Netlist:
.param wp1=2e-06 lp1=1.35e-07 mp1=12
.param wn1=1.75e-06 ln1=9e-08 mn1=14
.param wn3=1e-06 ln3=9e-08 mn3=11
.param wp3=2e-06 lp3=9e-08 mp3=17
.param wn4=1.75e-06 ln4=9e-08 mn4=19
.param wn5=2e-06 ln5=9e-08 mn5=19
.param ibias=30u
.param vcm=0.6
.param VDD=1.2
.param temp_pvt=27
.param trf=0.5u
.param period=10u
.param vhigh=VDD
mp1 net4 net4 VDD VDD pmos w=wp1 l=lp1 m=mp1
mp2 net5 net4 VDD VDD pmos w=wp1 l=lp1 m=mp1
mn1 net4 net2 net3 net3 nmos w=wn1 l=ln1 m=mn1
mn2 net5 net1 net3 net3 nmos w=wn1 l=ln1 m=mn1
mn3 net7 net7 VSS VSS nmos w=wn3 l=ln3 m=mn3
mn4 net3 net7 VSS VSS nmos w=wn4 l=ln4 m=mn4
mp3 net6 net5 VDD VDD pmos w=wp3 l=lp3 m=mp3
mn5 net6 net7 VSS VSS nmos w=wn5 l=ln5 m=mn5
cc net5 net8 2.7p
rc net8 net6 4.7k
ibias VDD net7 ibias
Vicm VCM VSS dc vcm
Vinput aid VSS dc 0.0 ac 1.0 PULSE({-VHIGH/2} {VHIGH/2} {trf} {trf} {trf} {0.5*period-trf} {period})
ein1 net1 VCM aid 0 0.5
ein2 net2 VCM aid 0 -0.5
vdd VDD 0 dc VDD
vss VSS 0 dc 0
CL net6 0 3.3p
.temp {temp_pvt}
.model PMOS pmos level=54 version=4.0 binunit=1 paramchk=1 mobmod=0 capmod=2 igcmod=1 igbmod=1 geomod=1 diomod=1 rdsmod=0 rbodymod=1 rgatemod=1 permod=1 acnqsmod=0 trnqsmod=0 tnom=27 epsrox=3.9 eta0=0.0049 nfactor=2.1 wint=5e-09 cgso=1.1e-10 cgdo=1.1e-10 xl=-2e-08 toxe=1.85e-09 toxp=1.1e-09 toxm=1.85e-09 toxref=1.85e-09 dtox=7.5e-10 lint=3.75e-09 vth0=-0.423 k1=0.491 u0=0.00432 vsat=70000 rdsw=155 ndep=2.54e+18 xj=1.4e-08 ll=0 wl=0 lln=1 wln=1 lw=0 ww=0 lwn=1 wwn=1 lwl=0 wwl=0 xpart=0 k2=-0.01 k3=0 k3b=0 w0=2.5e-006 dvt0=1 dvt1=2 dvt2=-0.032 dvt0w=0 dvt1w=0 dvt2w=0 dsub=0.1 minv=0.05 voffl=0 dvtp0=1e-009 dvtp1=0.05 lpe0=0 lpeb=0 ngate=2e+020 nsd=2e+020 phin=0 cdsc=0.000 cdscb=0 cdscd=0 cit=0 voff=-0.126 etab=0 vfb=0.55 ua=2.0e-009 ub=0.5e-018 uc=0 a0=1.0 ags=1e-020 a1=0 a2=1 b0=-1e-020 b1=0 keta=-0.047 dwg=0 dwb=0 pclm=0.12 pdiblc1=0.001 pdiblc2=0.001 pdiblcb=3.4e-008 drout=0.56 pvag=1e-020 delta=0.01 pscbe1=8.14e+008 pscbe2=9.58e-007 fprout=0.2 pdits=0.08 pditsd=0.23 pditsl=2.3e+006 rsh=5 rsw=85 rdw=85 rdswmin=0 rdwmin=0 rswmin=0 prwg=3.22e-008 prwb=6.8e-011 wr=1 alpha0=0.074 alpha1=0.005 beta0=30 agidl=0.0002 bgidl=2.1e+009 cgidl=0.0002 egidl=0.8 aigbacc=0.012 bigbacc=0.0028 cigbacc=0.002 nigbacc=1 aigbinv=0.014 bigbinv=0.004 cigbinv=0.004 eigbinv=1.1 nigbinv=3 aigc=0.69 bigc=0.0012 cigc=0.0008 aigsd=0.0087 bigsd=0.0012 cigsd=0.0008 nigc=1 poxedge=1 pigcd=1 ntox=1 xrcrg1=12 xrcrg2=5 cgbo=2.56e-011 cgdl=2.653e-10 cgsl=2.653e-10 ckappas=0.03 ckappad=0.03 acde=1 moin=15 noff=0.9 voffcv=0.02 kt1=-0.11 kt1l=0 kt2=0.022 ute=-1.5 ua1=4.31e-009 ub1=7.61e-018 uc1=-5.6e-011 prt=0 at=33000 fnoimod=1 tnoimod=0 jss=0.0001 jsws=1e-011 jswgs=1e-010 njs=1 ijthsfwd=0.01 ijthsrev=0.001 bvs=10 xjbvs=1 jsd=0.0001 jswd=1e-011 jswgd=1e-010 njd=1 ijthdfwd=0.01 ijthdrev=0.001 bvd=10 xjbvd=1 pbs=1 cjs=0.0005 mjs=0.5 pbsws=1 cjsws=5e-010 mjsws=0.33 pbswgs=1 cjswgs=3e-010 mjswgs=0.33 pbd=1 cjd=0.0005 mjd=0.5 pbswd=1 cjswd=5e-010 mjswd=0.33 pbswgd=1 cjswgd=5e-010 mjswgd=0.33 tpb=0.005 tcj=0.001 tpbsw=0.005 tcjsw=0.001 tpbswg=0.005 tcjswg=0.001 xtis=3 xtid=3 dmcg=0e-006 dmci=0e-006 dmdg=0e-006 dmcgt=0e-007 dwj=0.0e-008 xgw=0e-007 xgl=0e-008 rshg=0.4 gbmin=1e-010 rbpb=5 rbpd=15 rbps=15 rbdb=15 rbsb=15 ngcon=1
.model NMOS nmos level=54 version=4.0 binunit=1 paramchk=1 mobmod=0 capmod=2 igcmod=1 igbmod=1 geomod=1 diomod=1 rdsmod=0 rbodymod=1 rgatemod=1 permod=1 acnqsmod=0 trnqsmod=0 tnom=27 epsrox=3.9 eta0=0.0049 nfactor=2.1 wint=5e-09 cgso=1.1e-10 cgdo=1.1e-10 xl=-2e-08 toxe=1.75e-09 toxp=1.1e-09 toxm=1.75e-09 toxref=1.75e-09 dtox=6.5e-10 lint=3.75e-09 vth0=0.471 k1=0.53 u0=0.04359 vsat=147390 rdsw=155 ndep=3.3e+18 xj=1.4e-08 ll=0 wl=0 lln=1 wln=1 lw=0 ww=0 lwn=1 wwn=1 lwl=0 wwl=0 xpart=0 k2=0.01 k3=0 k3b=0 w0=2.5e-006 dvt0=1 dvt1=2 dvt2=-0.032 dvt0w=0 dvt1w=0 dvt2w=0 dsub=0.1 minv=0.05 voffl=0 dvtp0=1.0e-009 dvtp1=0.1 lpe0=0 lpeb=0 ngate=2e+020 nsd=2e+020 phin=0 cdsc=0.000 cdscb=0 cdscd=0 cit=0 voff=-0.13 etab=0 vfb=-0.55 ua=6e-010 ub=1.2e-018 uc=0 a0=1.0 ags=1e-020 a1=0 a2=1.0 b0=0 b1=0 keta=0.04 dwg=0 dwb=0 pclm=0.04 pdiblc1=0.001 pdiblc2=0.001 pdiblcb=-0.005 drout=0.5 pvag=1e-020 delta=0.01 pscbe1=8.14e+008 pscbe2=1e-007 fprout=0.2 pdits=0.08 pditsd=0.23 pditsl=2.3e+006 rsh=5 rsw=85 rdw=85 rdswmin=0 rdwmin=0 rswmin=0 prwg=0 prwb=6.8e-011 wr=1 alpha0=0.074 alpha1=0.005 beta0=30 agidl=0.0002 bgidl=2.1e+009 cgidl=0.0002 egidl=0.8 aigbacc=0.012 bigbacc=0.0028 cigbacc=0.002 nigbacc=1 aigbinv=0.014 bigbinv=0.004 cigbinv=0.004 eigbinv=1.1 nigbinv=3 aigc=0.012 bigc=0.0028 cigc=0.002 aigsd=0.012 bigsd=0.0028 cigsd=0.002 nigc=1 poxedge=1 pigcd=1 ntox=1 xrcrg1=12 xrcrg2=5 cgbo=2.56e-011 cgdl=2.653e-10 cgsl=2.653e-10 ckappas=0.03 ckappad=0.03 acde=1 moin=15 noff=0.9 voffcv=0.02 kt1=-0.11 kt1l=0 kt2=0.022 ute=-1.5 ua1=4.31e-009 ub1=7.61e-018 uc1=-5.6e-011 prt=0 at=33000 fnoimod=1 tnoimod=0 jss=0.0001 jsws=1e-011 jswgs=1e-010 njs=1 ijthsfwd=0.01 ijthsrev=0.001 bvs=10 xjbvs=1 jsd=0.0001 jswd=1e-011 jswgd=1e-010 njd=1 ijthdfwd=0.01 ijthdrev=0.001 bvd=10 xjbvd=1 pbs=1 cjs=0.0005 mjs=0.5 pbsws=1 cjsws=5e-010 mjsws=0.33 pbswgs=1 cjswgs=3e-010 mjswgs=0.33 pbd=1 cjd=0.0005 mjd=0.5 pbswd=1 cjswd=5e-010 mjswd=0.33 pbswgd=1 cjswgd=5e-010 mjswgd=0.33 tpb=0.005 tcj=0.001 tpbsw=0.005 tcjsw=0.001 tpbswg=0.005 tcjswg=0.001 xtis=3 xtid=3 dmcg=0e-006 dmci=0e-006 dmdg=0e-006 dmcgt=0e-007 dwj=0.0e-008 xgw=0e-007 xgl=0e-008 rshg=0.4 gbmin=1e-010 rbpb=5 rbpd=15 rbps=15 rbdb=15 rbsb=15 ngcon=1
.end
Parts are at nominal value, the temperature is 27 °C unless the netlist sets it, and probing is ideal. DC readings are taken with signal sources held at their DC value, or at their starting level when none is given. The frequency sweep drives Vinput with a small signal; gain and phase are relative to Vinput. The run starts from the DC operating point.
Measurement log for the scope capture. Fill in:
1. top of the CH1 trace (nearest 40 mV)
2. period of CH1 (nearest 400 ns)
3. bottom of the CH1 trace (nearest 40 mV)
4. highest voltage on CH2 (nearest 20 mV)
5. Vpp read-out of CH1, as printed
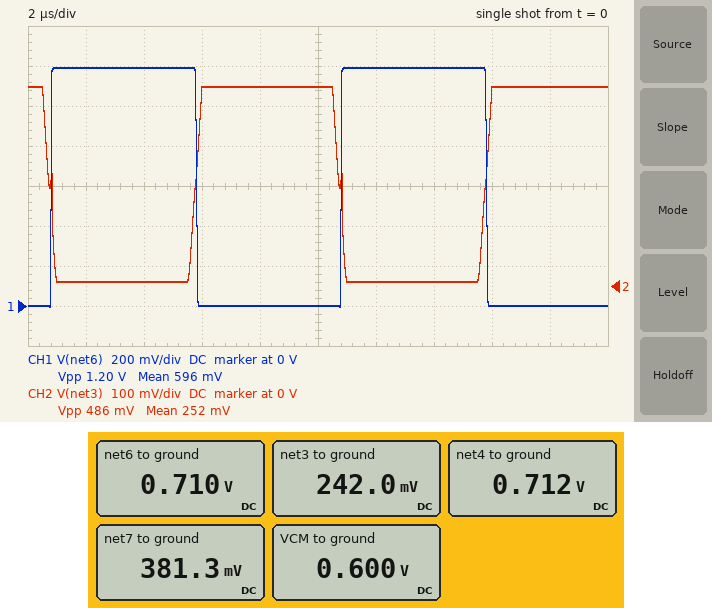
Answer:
1.20 V
10.0 µs
0 V
500 mV
1.20 V
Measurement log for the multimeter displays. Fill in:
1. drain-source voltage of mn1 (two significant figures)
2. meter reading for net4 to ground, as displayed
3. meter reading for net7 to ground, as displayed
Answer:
470 mV
0.712 V
381.3 mV
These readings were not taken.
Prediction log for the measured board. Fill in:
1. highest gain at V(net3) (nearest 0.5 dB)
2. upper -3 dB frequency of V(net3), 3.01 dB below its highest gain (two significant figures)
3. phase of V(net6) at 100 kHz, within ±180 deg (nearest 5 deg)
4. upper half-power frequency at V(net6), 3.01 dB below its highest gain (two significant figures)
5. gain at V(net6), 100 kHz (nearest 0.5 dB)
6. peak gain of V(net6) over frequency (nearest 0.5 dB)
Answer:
-9.0 dB
50 kHz
-65 deg
50 kHz
52.5 dB
59.5 dB
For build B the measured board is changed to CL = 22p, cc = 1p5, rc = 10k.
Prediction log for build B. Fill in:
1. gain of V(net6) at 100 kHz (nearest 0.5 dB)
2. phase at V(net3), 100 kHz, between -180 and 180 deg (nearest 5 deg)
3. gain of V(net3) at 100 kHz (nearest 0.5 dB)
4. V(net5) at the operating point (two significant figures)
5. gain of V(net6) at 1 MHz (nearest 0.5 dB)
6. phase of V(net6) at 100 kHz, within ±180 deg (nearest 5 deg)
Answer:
55.5 dB
140 deg
-13.0 dB
710 mV
37.5 dB
-50 deg
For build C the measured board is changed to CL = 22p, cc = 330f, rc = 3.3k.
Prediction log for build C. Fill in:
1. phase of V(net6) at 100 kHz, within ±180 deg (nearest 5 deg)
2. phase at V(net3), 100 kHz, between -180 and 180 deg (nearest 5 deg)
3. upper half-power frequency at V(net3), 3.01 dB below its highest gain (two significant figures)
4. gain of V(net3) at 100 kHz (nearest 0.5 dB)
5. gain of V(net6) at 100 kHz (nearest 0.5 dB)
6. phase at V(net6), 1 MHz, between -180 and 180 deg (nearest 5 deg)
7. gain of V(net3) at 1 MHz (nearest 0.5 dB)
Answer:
-25 deg
170 deg
310 kHz
-9.5 dB
59.0 dB
-80 deg
-15.0 dB
